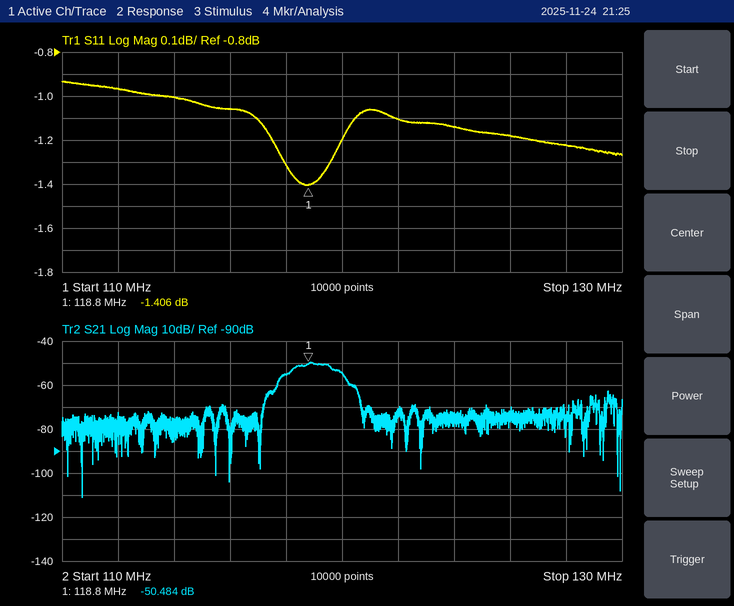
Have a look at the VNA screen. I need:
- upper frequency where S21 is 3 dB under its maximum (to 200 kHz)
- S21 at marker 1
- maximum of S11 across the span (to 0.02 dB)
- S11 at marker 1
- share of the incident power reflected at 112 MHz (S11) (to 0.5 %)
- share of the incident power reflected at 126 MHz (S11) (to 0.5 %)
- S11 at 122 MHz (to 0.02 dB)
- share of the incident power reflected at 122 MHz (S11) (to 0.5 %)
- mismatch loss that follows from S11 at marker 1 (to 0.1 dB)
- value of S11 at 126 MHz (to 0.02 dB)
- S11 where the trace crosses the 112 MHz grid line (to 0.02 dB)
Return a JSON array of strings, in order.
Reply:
["119.6 MHz", "-50.484 dB", "-0.94 dB", "-1.406 dB", "80.0 %", "76.0 %", "-1.10 dB", "77.5 %", "5.6 dB", "-1.18 dB", "-0.96 dB"]
